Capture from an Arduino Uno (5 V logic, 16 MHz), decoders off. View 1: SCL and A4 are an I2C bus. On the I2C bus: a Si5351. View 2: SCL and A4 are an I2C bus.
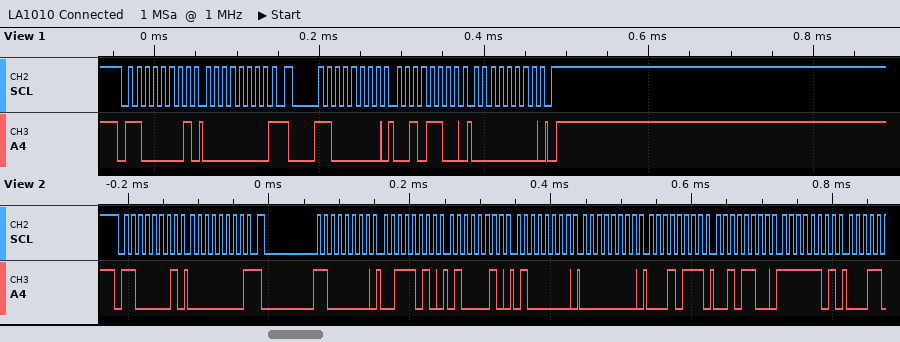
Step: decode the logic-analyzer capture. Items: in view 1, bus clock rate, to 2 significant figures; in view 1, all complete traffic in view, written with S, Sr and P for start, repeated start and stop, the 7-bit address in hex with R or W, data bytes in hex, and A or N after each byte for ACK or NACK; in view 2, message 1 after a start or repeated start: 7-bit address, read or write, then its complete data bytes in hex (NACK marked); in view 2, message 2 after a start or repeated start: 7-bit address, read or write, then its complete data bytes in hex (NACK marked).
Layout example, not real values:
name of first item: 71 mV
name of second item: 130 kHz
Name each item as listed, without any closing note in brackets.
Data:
in view 1, bus clock rate, to 2 significant figures: 100 kHz
in view 1, all complete traffic in view, written with S, Sr and P for start, repeated start and stop, the 7-bit address in hex with R or W, data bytes in hex, and A or N after each byte for ACK or NACK: S 60R A 00 N Sr 60W A 2C A 00 A P
in view 2, message 1 after a start or repeated start: 7-bit address, read or write, then its complete data bytes in hex: 0x60 read: 00 NACK
in view 2, message 2 after a start or repeated start: 7-bit address, read or write, then its complete data bytes in hex: 0x60 write: 3A 42 40 00 17 2C FD
